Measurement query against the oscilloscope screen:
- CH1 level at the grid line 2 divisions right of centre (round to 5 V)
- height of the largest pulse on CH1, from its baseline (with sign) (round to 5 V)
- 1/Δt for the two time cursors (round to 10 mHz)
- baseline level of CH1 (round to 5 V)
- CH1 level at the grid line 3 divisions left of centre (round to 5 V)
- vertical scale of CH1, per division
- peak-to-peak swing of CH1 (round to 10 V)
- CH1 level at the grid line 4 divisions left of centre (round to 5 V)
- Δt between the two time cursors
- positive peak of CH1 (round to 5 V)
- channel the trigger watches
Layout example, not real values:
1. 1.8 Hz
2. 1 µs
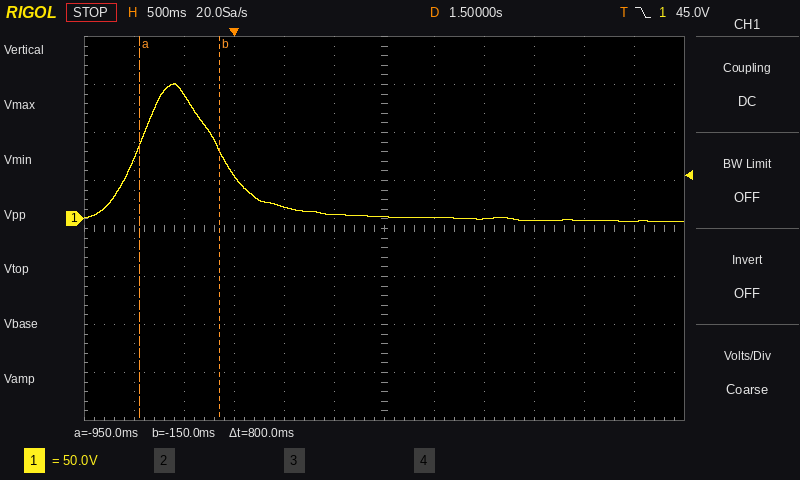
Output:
1. 0 V
2. +140 V
3. 1.25 Hz
4. 0 V
5. 45 V
6. 50 V
7. 140 V
8. 130 V
9. 800 ms
10. 140 V
11. CH1
